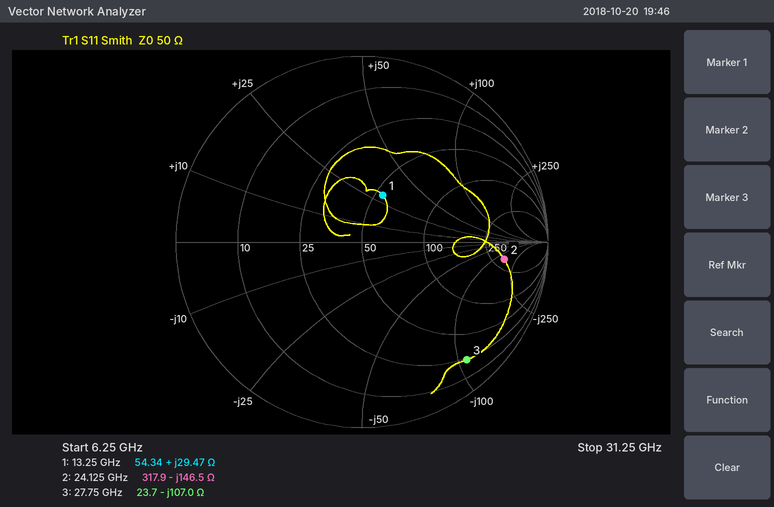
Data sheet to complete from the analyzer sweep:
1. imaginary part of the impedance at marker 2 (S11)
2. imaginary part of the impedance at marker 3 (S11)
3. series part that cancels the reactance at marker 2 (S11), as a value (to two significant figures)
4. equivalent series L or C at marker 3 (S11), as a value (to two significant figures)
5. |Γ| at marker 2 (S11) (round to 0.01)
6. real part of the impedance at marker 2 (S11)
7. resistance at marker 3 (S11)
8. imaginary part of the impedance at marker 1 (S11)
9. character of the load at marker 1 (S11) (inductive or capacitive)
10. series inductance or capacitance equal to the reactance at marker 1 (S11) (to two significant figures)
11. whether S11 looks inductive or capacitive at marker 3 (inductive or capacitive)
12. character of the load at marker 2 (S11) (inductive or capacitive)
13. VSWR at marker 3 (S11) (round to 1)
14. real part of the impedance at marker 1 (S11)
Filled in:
-146.5 Ω
-107.0 Ω
970 pH
54 fF
0.77
317.9 Ω
23.7 Ω
+29.47 Ω
inductive
350 pH
capacitive
capacitive
12
54.34 Ω
